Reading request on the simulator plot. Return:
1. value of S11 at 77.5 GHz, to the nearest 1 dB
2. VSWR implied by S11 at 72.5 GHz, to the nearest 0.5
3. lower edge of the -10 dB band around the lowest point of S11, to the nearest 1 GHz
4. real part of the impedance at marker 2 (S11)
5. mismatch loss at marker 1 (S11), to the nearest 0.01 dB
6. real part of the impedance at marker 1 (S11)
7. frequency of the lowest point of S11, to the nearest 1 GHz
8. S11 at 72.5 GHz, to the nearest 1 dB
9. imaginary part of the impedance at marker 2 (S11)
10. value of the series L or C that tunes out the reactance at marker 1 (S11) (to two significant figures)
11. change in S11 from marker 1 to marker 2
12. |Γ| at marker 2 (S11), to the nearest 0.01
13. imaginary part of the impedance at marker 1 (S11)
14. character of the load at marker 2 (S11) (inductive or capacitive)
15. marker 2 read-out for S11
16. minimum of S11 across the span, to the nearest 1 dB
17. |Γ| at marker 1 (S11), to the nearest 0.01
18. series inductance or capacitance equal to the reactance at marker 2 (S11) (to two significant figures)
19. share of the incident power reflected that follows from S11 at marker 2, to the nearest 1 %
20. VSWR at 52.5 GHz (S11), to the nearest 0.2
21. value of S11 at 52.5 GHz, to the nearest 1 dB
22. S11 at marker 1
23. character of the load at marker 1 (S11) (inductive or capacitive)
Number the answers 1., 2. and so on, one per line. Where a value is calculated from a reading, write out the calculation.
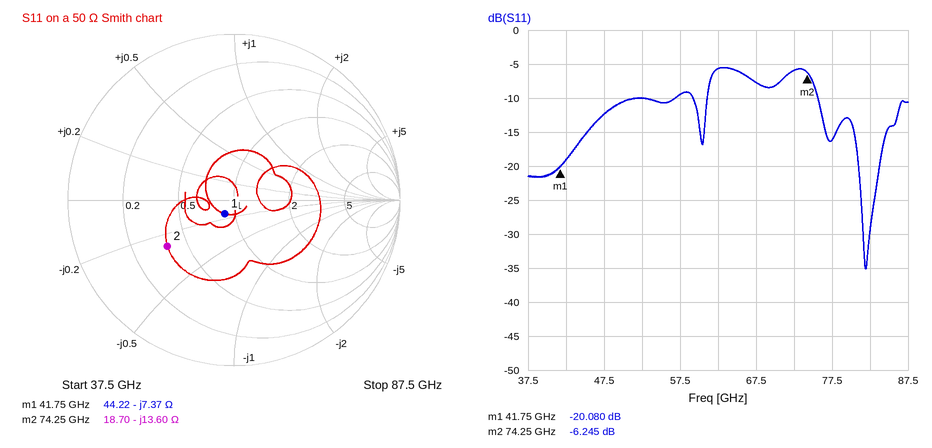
1. -16 dB
2. |Γ| = 10^(-6/20) = 0.5012; VSWR = (1 + 0.5012)/(1 − 0.5012) ≈ 3.0
3. 76 GHz
4. 18.70 Ω
5. −10 log10(1 − 10^(-20.08/10)) ≈ 0.04 dB
6. 44.22 Ω
7. 82 GHz
8. -6 dB
9. -13.60 Ω
10. L = 7.37 Ω/(2π × 41.75 GHz) ≈ 28 pH
11. -6.245 − (-20.08) = 13.835 dB
12. 0.49
13. -7.37 Ω
14. capacitive
15. -6.245 dB
16. -35 dB
17. 0.10
18. C = 1/(2π × 74.25 GHz × 13.6 Ω) ≈ 158 fF, so 160 fF to two significant figures
19. 10^(-6.245/10) ≈ 24 %
20. |Γ| = 10^(-10/20) = 0.3162; VSWR = (1 + 0.3162)/(1 − 0.3162) ≈ 1.92, so 2.0 to the nearest 0.2
21. -10 dB
22. -20.080 dB
23. capacitive
